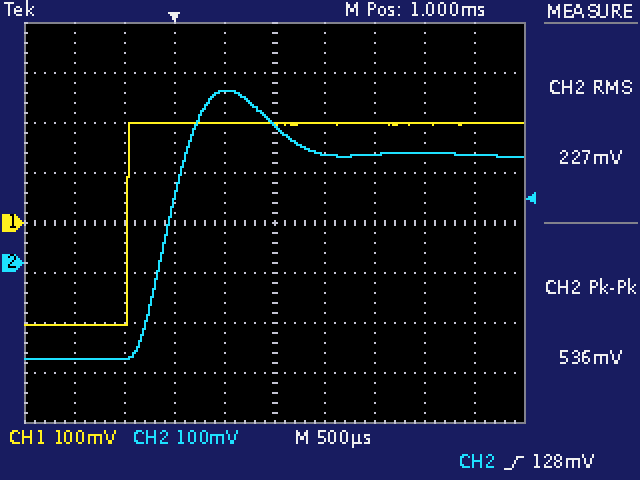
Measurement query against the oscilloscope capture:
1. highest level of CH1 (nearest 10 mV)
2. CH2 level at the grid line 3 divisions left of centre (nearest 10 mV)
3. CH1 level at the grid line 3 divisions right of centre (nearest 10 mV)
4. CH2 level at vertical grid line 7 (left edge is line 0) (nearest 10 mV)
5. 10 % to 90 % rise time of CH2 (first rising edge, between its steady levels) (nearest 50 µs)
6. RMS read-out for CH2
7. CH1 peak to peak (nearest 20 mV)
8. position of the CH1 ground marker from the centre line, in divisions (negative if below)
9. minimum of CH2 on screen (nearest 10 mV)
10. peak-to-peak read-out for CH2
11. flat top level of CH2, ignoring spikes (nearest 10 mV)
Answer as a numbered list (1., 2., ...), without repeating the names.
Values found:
1. 200 mV
2. -190 mV
3. 200 mV
4. 220 mV
5. 400 µs
6. 227 mV
7. 400 mV
8. 0.0 div
9. -190 mV
10. 536 mV
11. 220 mV
